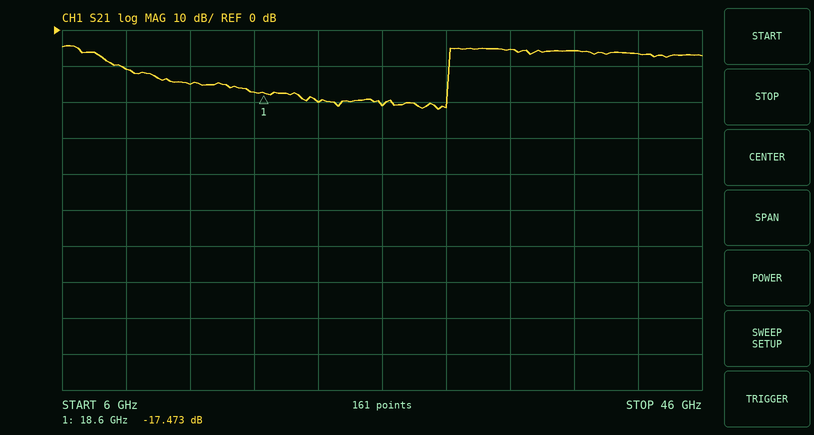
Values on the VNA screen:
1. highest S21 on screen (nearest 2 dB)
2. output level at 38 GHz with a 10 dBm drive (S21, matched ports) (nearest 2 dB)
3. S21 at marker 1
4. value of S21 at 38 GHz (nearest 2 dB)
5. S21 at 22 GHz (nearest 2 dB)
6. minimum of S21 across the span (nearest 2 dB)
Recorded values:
-4 dB
4 dBm
-17.473 dB
-6 dB
-20 dB
-22 dB
